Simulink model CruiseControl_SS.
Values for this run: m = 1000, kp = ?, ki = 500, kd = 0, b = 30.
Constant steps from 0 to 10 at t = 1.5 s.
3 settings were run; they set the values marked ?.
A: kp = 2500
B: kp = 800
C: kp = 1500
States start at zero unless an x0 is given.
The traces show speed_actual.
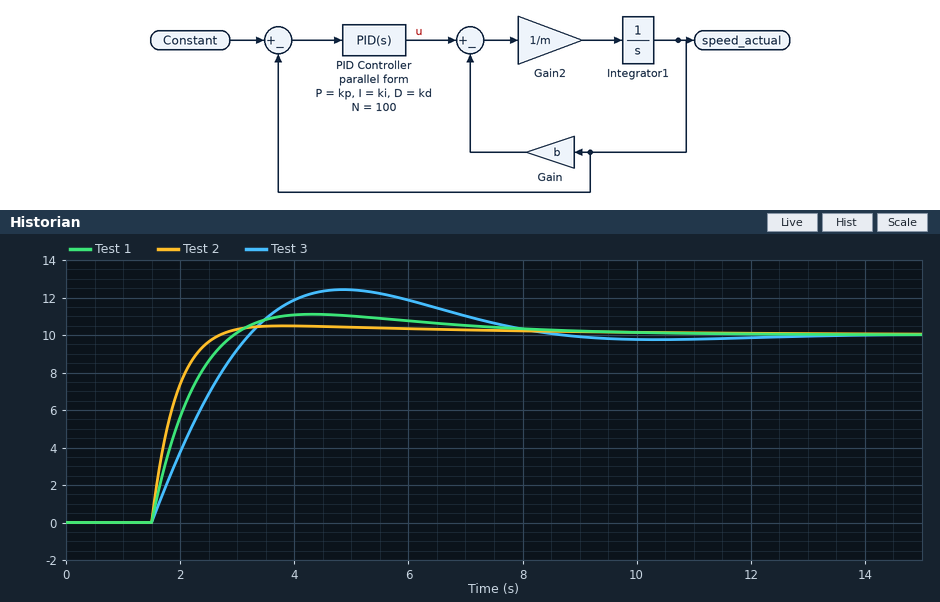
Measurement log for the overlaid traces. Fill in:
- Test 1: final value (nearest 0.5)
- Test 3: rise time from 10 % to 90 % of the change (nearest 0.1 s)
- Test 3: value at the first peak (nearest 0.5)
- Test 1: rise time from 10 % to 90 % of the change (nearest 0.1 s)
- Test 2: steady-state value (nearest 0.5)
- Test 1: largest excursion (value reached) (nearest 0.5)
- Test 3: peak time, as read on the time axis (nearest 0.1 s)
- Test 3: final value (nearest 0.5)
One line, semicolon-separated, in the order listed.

10.0; 1.3 s; 12.5; 1.0 s; 10.0; 11.0; 4.9 s; 10.0
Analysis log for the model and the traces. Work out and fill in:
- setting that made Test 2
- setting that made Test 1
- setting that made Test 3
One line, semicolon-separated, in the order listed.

A; C; B
